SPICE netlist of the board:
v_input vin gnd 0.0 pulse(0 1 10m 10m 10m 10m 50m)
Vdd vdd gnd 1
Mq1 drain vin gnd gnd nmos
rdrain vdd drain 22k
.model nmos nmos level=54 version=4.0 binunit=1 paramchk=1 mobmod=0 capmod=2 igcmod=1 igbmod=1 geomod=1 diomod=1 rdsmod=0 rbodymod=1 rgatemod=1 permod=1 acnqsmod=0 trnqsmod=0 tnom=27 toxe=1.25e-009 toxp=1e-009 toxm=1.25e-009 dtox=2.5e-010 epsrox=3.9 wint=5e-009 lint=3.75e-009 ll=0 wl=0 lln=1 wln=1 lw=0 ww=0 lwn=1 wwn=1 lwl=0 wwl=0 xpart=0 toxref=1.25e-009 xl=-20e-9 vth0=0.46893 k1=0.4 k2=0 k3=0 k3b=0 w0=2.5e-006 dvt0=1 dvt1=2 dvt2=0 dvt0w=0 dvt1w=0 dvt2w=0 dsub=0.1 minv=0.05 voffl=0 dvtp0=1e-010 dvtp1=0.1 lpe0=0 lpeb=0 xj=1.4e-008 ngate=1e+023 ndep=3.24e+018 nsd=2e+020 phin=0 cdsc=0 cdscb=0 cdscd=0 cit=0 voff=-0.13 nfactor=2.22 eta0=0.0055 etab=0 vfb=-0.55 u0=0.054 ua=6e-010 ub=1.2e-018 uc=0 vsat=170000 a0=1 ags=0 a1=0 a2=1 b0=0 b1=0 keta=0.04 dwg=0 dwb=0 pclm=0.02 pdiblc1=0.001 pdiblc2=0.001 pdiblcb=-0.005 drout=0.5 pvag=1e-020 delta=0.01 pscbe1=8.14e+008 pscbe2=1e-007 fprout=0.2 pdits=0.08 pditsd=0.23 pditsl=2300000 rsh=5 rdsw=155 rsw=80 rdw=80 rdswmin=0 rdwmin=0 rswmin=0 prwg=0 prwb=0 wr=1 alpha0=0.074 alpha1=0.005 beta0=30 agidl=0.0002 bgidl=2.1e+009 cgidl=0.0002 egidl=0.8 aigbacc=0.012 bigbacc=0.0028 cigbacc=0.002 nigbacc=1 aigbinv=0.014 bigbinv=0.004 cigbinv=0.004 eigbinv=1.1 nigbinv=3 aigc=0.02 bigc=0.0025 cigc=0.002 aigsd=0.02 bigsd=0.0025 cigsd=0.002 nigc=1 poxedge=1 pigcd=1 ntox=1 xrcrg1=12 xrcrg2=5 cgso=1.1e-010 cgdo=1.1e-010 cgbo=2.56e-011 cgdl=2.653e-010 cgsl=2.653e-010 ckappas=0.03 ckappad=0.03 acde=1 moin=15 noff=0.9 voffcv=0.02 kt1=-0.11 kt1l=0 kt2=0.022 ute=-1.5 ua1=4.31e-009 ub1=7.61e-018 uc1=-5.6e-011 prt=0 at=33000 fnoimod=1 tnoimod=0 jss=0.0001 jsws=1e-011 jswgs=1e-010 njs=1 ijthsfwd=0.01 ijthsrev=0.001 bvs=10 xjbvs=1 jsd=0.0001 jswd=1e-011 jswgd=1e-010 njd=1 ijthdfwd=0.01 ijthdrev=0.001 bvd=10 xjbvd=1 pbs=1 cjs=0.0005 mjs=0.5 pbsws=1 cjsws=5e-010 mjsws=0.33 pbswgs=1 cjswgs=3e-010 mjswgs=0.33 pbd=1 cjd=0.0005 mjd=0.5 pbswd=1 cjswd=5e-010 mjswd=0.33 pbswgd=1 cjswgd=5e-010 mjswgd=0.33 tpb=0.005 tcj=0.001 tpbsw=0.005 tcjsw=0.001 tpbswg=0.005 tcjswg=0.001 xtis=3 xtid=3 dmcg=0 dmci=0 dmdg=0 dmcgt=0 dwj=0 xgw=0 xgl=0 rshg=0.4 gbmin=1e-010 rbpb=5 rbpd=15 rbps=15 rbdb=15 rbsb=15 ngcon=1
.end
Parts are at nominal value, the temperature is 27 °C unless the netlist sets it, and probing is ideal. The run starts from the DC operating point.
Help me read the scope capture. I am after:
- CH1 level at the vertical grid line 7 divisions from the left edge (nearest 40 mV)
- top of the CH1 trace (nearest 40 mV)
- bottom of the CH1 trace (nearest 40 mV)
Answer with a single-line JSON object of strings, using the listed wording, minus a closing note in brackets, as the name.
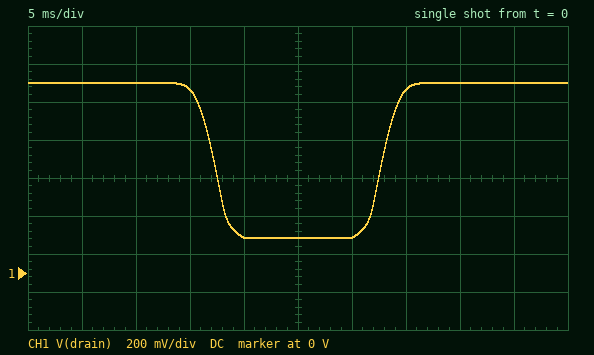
{"CH1 level at the vertical grid line 7 divisions from the left edge": "960 mV", "top of the CH1 trace": "1.00 V", "bottom of the CH1 trace": "200 mV"}
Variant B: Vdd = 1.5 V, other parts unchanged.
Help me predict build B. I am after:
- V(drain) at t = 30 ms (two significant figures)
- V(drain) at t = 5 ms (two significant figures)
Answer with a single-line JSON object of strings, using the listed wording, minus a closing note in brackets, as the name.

{"V(drain) at t = 30 ms": "330 mV", "V(drain) at t = 5 ms": "1.5 V"}
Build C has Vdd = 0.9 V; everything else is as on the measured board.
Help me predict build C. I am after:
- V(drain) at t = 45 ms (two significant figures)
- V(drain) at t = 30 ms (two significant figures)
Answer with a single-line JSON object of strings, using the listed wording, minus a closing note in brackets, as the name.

{"V(drain) at t = 45 ms": "900 mV", "V(drain) at t = 30 ms": "160 mV"}
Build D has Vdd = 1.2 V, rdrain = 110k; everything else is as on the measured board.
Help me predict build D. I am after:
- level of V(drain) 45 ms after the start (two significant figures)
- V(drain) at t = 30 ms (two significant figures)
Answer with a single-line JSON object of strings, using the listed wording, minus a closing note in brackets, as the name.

{"level of V(drain) 45 ms after the start": "1.2 V", "V(drain) at t = 30 ms": "45 mV"}
